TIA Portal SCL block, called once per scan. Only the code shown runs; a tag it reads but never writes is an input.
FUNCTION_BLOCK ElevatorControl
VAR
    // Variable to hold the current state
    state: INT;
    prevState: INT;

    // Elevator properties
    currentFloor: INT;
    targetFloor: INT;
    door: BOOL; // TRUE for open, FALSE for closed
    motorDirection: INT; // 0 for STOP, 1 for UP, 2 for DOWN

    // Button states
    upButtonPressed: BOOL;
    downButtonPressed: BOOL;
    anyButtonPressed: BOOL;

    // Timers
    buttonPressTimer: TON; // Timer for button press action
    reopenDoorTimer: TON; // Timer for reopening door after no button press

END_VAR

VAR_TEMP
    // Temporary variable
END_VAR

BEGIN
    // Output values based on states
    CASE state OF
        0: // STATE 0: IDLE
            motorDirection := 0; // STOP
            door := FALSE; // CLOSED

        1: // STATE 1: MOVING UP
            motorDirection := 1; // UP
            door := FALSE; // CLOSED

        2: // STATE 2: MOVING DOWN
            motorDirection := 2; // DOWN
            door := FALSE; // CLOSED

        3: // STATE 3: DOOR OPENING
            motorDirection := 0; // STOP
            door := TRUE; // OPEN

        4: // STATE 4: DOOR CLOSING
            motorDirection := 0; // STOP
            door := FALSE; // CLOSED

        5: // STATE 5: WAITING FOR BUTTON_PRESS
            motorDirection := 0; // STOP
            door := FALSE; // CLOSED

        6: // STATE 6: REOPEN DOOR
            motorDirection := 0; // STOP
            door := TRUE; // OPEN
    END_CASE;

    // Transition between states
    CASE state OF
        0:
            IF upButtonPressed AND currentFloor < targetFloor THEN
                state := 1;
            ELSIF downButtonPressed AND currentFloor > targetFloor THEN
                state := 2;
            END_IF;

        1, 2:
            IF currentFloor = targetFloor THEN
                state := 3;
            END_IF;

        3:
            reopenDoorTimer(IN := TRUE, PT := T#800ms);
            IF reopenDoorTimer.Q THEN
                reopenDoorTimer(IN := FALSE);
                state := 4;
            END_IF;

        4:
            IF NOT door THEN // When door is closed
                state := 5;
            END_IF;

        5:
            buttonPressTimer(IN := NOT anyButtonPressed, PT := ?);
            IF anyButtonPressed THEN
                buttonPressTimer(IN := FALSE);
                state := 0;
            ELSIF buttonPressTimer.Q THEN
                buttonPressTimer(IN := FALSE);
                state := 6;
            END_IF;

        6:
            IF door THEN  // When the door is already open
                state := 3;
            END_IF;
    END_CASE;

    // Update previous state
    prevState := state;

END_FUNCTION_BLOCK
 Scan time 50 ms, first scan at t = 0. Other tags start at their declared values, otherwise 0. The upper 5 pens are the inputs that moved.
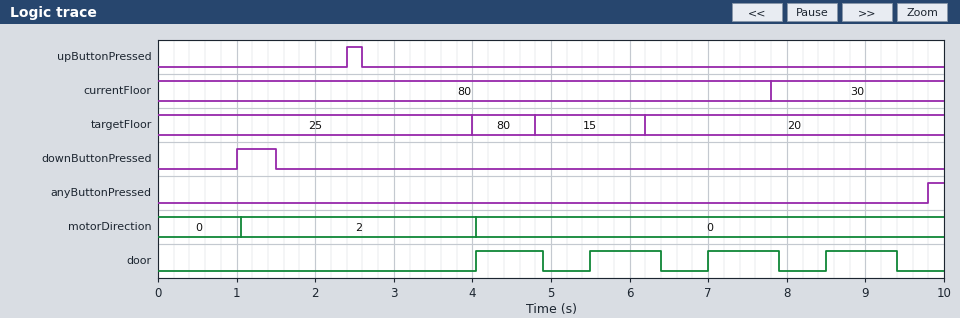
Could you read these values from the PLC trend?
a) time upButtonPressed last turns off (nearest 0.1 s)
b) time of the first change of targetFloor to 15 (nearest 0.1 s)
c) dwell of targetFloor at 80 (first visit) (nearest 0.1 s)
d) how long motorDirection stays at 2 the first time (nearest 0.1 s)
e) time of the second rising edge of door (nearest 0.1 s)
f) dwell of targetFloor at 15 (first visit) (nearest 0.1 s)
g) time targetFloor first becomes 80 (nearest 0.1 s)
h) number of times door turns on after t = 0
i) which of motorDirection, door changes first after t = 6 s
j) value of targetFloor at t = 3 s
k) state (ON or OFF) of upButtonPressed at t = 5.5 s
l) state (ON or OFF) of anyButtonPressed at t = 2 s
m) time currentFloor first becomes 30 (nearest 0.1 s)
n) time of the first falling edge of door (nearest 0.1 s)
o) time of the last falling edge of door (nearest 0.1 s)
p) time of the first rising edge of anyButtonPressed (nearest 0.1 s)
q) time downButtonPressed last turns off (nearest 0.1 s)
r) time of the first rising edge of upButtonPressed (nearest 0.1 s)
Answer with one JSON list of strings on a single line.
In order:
["2.6 s", "4.8 s", "0.8 s", "3.0 s", "5.5 s", "1.4 s", "4.0 s", "4", "door", "25", "OFF", "OFF", "7.8 s", "4.9 s", "9.4 s", "9.8 s", "1.5 s", "2.4 s"]
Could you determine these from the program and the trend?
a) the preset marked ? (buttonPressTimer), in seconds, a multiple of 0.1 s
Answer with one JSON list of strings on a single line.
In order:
["0.5 s"]
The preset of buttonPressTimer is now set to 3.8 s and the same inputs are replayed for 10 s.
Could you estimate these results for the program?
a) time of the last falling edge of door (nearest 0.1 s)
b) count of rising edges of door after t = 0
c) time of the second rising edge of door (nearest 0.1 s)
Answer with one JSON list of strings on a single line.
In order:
["9.7 s", "2", "8.8 s"]
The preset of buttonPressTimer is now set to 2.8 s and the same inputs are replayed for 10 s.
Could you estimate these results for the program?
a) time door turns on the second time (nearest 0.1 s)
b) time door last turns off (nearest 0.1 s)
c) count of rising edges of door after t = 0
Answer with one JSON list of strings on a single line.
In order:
["7.8 s", "8.7 s", "2"]
